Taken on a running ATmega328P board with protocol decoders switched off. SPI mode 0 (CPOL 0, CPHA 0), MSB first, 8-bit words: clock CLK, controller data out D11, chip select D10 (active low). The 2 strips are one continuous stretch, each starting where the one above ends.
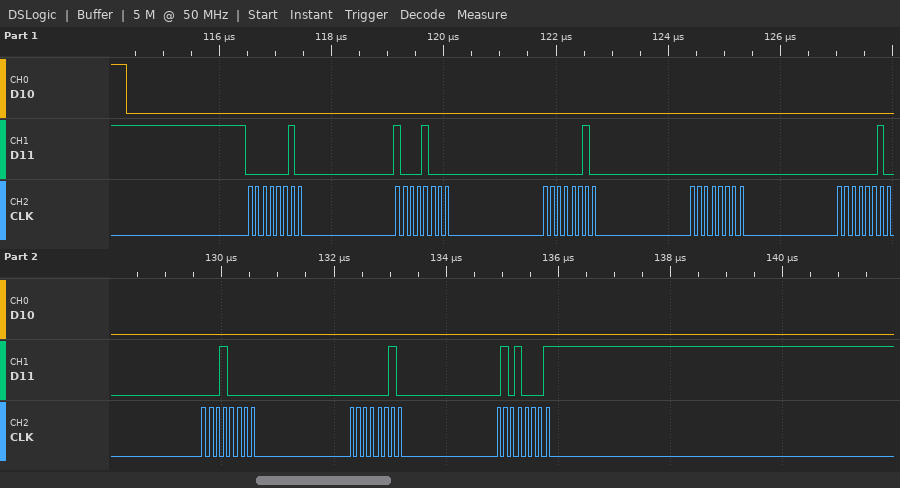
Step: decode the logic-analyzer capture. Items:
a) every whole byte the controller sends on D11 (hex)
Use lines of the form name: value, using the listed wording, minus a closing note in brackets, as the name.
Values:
every whole byte the controller sends on D11: 02 88 02 00 02 10 02 51
